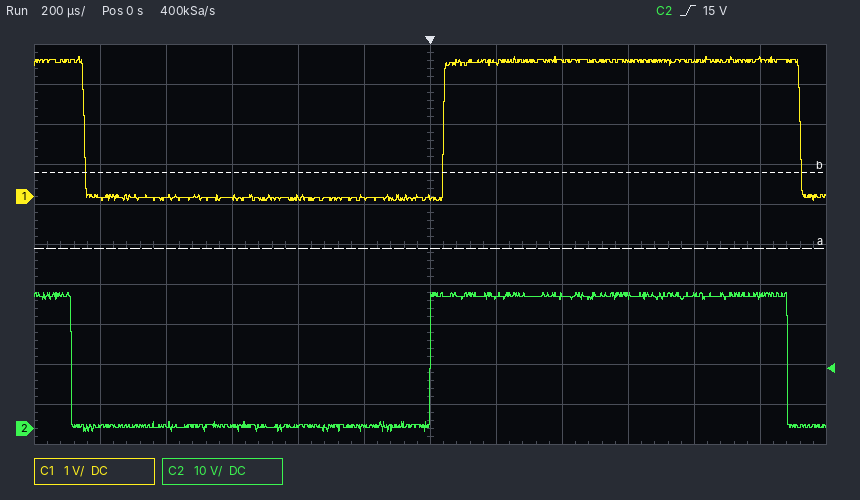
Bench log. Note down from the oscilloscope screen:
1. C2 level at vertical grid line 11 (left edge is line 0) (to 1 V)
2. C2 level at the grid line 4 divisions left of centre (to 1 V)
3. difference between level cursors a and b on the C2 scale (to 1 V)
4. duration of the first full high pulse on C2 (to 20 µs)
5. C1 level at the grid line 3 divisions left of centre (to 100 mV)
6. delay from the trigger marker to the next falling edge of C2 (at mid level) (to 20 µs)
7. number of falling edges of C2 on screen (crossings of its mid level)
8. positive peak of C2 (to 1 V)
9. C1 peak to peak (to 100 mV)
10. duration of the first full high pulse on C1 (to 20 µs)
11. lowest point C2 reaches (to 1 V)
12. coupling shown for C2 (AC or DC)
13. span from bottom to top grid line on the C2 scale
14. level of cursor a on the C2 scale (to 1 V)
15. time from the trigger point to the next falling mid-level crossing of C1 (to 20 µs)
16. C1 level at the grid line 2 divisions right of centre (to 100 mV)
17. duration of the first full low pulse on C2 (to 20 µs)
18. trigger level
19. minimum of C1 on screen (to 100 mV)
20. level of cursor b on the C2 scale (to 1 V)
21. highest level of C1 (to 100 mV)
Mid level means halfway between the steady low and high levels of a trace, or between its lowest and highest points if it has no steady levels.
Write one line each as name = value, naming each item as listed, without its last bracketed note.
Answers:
C2 level at vertical grid line 11 (left edge is line 0) = 33 V
C2 level at the grid line 4 divisions left of centre = 1 V
difference between level cursors a and b on the C2 scale = 19 V
duration of the first full high pulse on C2 = 1.08 ms
C1 level at the grid line 3 divisions left of centre = 0.0 V
delay from the trigger marker to the next falling edge of C2 (at mid level) = 1.08 ms
number of falling edges of C2 on screen = 2
positive peak of C2 = 34 V
C1 peak to peak = 3.6 V
duration of the first full high pulse on C1 = 1.08 ms
lowest point C2 reaches = -1 V
coupling shown for C2 = DC
span from bottom to top grid line on the C2 scale = 100 V
level of cursor a on the C2 scale = 45 V
time from the trigger point to the next falling mid-level crossing of C1 = 1.12 ms
C1 level at the grid line 2 divisions right of centre = 3.4 V
duration of the first full low pulse on C2 = 1.08 ms
trigger level = 15 V
minimum of C1 on screen = -100 mV
level of cursor b on the C2 scale = 64 V
highest level of C1 = 3.5 V
